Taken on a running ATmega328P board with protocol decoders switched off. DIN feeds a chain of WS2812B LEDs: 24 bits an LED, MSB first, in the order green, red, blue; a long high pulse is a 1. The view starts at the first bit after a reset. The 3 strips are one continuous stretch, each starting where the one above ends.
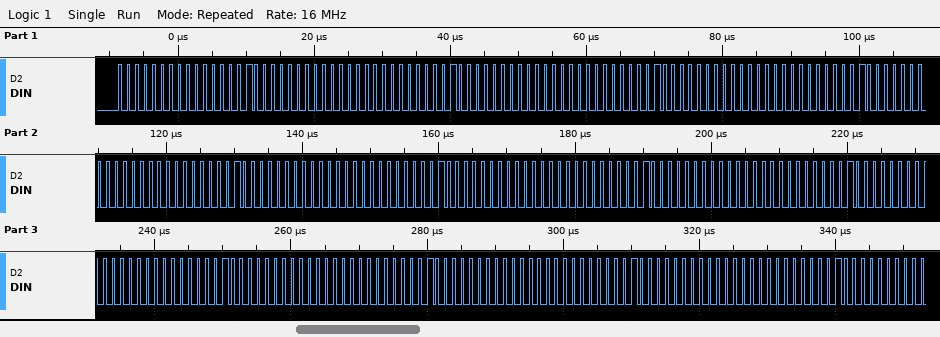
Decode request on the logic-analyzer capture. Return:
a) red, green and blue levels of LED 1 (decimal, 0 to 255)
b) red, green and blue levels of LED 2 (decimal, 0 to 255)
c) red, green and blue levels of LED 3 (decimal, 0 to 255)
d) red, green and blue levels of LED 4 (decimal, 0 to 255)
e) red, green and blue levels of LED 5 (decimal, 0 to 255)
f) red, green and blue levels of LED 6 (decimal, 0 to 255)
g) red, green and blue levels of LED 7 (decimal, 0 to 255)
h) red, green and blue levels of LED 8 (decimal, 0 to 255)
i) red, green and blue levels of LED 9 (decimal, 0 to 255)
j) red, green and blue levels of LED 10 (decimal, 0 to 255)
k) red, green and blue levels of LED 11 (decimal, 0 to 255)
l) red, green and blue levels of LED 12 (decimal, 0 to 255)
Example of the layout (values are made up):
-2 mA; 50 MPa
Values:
1, 0, 0; 1, 0, 0; 1, 0, 0; 1, 0, 0; 1, 0, 0; 1, 0, 0; 1, 0, 0; 1, 0, 0; 1, 0, 0; 1, 0, 0; 1, 0, 0; 1, 0, 0
